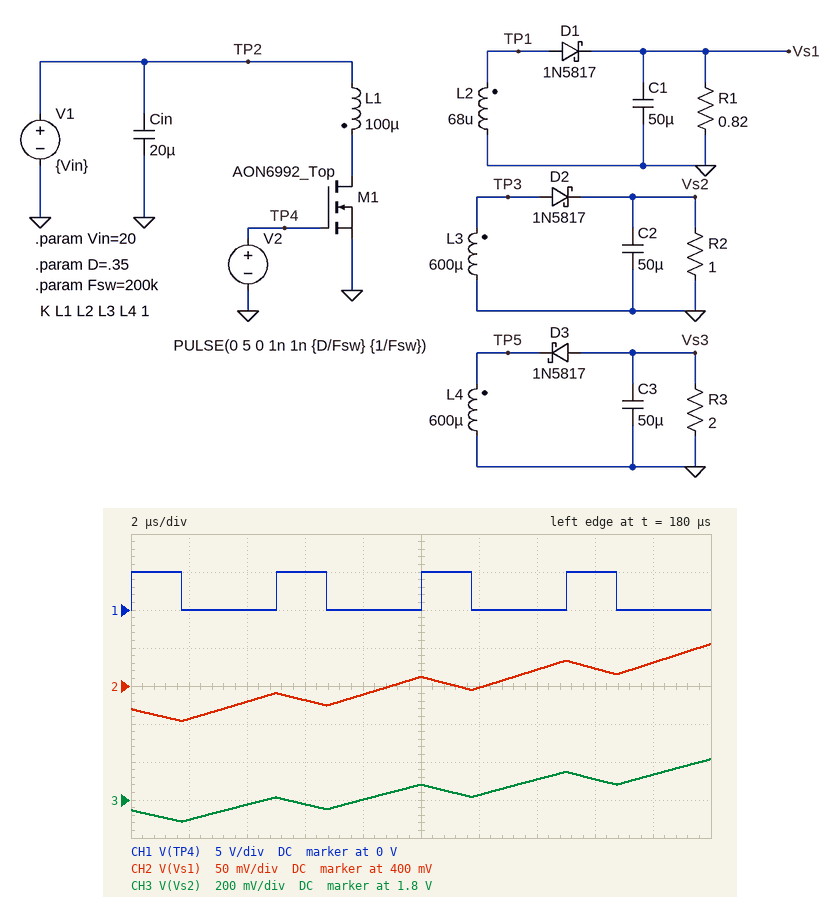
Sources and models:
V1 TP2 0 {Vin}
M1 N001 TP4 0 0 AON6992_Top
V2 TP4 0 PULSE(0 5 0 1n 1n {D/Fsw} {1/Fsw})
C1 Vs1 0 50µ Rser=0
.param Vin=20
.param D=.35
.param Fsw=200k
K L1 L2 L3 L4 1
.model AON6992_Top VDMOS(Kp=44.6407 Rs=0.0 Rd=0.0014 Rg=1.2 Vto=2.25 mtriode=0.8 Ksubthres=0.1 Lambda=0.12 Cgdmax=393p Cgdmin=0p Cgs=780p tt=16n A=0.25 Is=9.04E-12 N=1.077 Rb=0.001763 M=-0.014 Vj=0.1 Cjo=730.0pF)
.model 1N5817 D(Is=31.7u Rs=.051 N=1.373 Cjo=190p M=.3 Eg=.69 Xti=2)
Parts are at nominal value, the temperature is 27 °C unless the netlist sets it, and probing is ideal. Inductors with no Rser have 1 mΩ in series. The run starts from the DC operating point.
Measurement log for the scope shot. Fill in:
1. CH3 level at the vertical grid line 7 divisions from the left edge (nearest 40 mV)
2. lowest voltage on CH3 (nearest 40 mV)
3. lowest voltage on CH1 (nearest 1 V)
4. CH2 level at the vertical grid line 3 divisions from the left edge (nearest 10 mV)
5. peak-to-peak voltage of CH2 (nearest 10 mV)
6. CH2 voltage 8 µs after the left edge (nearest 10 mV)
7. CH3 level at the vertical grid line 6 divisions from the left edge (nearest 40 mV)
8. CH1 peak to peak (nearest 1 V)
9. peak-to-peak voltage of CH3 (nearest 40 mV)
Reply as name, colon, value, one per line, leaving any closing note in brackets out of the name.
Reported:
CH3 level at the vertical grid line 7 divisions from the left edge: 1.92 V
lowest voltage on CH3: 1.68 V
lowest voltage on CH1: 0 V
CH2 level at the vertical grid line 3 divisions from the left edge: 380 mV
peak-to-peak voltage of CH2: 100 mV
CH2 voltage 8 µs after the left edge: 390 mV
CH3 level at the vertical grid line 6 divisions from the left edge: 1.84 V
CH1 peak to peak: 5 V
peak-to-peak voltage of CH3: 320 mV
